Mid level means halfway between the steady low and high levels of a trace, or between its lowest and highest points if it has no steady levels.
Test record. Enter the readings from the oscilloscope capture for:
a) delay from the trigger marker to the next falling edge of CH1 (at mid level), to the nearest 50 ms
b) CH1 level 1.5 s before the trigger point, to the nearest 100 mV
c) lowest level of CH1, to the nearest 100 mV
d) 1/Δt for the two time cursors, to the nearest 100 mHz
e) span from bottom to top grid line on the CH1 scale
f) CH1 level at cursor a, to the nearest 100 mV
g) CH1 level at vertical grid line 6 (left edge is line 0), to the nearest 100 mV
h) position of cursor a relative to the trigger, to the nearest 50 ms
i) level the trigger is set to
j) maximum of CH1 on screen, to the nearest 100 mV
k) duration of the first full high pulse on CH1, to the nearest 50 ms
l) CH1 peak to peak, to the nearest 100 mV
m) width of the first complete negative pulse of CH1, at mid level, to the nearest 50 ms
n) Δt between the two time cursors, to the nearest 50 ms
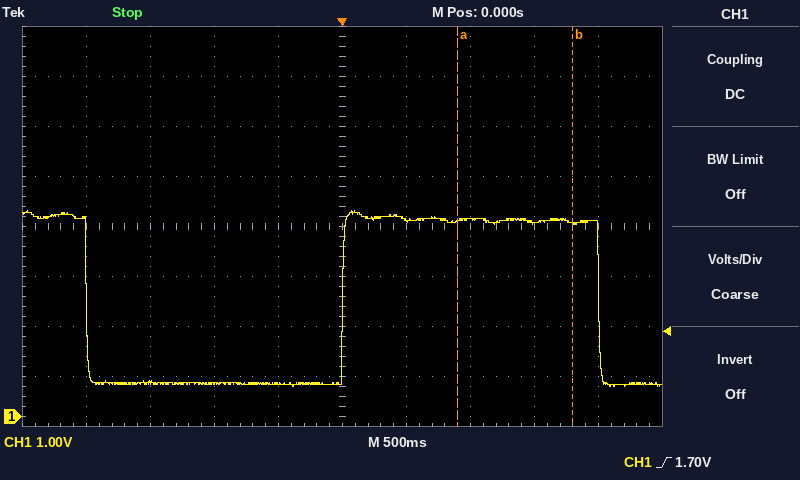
2.00 s
700 mV
600 mV
1.1 Hz
8 V
3.9 V
3.9 V
+900 ms
1.70 V
4.1 V
2.00 s
3.5 V
2.00 s
900 ms
